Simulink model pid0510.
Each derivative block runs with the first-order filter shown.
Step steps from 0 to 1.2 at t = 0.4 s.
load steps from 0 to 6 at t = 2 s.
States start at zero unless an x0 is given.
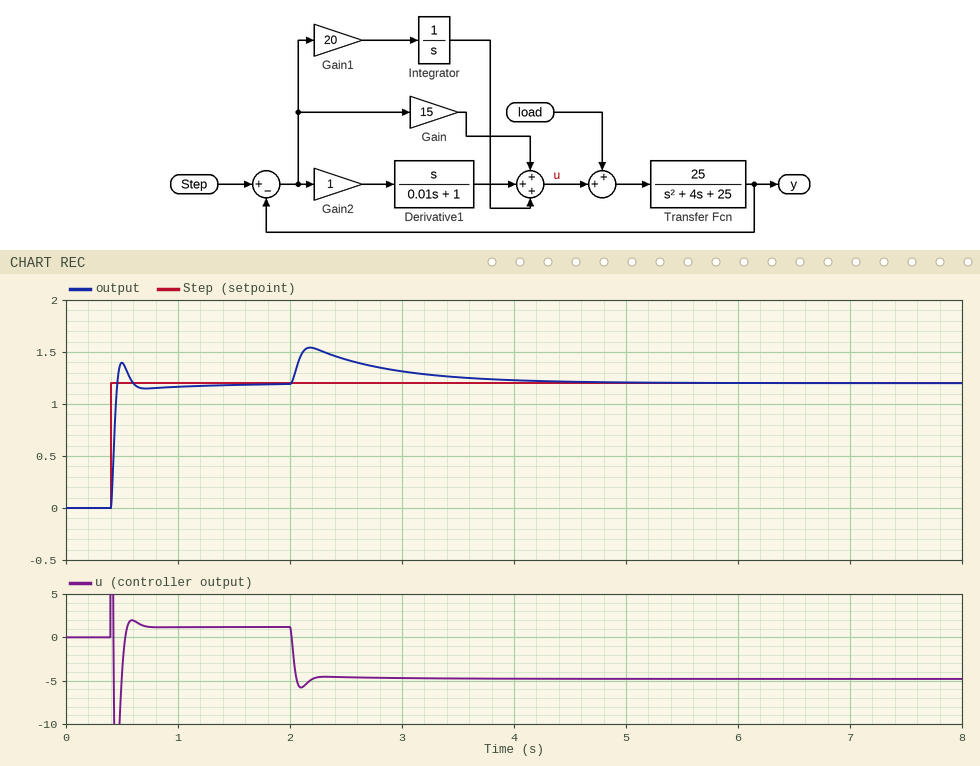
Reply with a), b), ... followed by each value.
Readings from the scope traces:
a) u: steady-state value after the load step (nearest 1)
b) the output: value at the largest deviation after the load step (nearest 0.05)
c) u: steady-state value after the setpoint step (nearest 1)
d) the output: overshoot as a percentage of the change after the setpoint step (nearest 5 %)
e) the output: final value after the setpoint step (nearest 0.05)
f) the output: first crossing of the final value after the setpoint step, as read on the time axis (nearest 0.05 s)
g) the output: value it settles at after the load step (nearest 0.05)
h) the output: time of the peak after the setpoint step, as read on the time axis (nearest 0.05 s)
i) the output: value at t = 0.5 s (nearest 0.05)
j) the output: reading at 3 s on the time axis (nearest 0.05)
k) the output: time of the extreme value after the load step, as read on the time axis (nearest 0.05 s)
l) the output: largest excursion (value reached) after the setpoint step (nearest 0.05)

a) -5
b) 1.55
c) 1
d) 15 %
e) 1.20
f) 0.45 s
g) 1.20
h) 0.50 s
i) 1.40
j) 1.30
k) 2.20 s
l) 1.40
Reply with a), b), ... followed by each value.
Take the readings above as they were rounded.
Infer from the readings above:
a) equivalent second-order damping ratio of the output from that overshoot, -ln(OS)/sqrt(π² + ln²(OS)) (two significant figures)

a) 0.52
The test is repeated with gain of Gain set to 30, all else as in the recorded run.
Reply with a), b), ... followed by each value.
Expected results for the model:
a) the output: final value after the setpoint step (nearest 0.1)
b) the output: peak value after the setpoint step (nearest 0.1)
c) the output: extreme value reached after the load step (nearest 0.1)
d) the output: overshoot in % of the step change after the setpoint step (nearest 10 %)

a) 1.2
b) 1.6
c) 1.4
d) 30 %
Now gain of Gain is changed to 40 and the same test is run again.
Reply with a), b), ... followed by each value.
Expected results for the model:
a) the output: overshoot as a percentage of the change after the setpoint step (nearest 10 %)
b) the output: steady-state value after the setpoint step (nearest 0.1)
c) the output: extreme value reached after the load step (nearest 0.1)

a) 40 %
b) 1.2
c) 1.4
